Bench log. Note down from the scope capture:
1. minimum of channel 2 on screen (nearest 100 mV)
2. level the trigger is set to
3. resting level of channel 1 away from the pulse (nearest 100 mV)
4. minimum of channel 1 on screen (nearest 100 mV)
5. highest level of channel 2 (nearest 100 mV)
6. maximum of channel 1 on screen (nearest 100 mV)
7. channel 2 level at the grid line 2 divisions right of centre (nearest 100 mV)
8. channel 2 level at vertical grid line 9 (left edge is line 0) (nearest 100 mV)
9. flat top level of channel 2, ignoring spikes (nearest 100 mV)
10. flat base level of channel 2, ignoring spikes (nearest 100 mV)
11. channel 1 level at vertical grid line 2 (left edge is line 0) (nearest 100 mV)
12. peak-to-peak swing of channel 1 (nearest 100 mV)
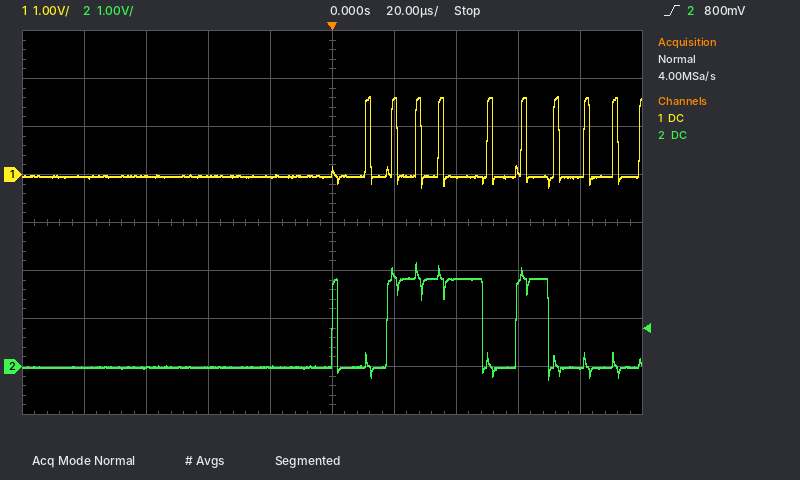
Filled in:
-300 mV
800 mV
0.0 V
-300 mV
2.2 V
1.6 V
1.8 V
0.0 V
1.8 V
0.0 V
0.0 V
1.9 V
